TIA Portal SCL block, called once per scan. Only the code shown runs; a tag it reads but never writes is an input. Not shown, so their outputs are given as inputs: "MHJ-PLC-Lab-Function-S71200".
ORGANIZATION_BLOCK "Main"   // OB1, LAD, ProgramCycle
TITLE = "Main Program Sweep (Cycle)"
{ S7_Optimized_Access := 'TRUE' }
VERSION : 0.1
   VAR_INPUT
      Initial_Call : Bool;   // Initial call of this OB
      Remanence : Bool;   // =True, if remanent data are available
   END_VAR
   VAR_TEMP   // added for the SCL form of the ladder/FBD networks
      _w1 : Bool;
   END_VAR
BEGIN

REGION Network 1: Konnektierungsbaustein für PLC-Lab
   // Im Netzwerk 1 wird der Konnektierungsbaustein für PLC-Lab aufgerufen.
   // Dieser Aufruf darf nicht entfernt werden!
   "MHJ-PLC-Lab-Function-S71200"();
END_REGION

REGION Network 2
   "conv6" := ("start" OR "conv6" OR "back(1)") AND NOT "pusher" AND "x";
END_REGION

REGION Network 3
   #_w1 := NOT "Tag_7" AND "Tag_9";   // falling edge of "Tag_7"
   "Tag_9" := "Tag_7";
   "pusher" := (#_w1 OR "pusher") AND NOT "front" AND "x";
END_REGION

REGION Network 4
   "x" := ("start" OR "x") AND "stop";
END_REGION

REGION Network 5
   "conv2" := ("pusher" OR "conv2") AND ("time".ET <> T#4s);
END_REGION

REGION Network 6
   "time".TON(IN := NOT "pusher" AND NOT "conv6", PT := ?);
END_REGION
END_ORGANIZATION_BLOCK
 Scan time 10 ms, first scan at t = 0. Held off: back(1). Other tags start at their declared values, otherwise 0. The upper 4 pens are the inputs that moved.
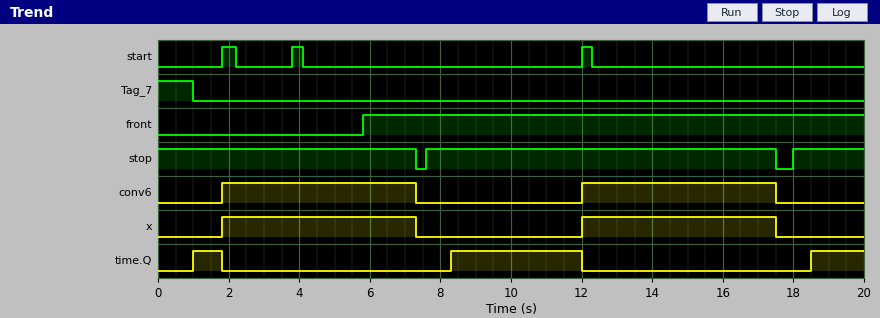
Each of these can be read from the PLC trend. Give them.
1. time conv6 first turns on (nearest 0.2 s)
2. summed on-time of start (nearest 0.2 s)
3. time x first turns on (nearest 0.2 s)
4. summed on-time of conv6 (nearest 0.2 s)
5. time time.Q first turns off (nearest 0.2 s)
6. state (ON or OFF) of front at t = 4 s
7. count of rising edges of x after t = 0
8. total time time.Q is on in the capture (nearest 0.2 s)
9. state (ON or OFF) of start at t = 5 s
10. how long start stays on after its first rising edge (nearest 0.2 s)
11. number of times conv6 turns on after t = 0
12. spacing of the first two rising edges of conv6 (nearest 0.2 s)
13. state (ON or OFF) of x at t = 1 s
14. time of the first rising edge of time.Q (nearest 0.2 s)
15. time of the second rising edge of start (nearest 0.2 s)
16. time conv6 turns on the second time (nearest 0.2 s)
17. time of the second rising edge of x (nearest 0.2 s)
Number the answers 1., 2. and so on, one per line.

1. 1.8 s
2. 1.0 s
3. 1.8 s
4. 11.0 s
5. 1.8 s
6. OFF
7. 2
8. 6.0 s
9. OFF
10. 0.4 s
11. 2
12. 10.2 s
13. OFF
14. 1.0 s
15. 3.8 s
16. 12.0 s
17. 12.0 s
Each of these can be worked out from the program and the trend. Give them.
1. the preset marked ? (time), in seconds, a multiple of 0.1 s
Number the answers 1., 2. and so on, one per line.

1. 1.0 s
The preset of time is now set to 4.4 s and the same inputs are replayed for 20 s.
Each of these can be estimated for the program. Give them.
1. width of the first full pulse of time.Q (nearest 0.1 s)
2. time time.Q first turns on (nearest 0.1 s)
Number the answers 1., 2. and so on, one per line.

1. 0.3 s
2. 11.7 s
